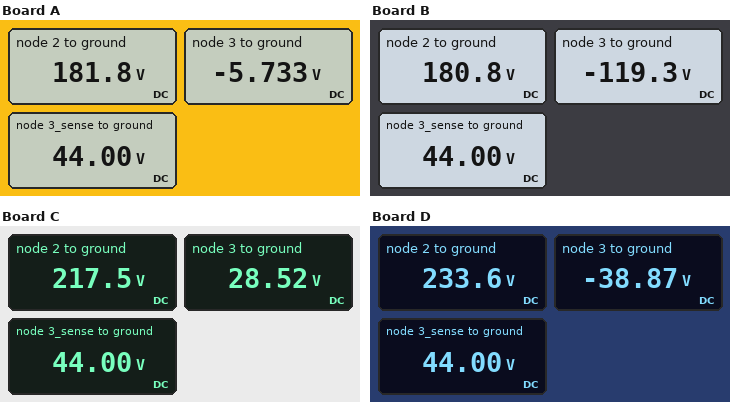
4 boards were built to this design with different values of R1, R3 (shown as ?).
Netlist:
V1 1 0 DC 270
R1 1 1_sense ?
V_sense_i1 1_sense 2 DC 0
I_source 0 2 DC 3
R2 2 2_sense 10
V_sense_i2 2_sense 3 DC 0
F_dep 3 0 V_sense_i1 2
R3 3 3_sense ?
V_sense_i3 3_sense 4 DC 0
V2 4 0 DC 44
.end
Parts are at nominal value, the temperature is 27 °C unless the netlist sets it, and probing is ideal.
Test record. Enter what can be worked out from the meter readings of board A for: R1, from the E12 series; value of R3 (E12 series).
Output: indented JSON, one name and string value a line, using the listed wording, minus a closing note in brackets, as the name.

{
  "R1, from the E12 series": "5.6 Ω",
  "value of R3": "3.9 Ω"
}
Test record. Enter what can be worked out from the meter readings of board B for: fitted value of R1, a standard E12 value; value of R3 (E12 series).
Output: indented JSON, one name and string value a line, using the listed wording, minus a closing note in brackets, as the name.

{
  "fitted value of R1, a standard E12 value": "3.3 Ω",
  "value of R3": "6.8 Ω"
}
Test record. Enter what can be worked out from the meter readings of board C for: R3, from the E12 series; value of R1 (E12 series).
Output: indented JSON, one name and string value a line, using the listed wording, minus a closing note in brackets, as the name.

{
  "R3, from the E12 series": "1.2 Ω",
  "value of R1": "3.3 Ω"
}
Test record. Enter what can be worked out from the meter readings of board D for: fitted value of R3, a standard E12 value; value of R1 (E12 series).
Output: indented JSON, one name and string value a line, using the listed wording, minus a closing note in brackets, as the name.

{
  "fitted value of R3, a standard E12 value": "3.9 Ω",
  "value of R1": "1.5 Ω"
}
